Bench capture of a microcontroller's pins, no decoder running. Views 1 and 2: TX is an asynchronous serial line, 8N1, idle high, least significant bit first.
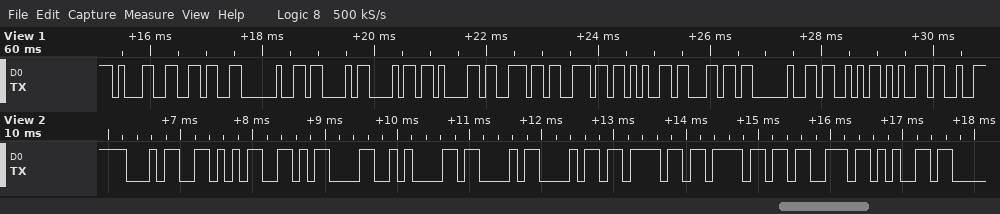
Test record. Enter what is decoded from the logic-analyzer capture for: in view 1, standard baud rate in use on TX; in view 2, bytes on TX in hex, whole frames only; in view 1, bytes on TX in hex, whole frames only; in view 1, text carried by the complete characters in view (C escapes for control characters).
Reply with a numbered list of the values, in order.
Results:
1. 9600 baud
2. 34 35 0D 0A 43 68 6F 6F 73 65
3. 0x31 0x36 0x20 0x43 0x68 0x61 0x6E 0x6E 0x65 0x6C 0x20 0x53 0x65
4. "16 Channel Se"
